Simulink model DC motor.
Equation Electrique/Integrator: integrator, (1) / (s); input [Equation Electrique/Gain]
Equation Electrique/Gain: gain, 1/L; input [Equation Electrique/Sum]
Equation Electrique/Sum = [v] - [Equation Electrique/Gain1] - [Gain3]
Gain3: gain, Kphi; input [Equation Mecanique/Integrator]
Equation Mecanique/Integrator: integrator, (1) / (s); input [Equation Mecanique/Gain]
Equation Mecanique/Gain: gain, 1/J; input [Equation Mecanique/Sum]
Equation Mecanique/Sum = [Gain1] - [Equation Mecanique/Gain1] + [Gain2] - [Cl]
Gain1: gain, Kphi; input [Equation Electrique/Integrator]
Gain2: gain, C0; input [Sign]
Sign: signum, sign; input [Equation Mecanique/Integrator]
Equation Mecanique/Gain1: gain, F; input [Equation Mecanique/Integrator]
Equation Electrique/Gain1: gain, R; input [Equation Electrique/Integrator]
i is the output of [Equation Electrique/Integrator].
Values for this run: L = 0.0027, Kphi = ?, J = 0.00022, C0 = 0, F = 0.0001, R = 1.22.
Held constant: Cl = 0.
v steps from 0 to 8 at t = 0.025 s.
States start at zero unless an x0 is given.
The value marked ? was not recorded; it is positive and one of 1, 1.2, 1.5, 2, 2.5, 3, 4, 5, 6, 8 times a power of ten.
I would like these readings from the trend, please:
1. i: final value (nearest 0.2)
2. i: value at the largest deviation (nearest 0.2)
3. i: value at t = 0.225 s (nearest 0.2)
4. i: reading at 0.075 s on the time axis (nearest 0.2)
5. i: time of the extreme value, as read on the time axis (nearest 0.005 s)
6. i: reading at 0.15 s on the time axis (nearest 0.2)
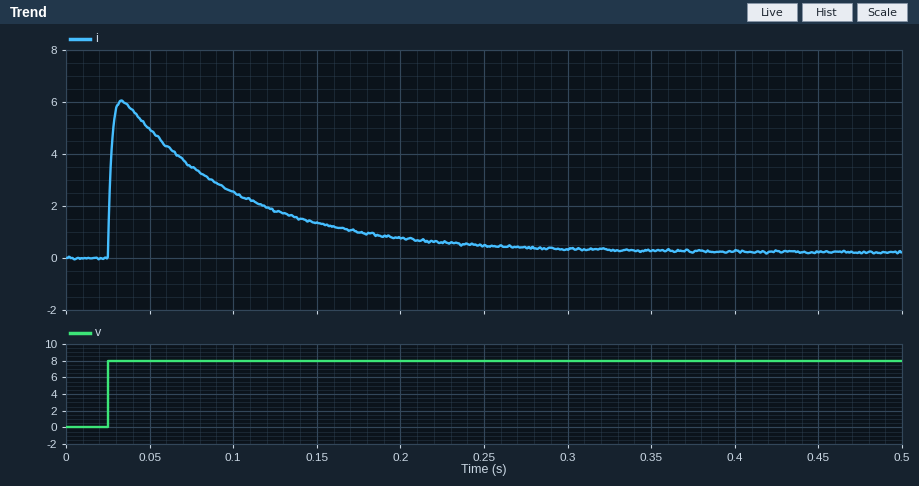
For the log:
0.2
6.0
0.6
3.6
0.035 s
1.4
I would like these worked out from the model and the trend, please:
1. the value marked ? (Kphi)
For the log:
0.06
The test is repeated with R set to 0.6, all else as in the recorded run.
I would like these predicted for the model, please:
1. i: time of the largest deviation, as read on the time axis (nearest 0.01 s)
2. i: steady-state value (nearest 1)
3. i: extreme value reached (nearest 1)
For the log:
0.04 s
0
11
